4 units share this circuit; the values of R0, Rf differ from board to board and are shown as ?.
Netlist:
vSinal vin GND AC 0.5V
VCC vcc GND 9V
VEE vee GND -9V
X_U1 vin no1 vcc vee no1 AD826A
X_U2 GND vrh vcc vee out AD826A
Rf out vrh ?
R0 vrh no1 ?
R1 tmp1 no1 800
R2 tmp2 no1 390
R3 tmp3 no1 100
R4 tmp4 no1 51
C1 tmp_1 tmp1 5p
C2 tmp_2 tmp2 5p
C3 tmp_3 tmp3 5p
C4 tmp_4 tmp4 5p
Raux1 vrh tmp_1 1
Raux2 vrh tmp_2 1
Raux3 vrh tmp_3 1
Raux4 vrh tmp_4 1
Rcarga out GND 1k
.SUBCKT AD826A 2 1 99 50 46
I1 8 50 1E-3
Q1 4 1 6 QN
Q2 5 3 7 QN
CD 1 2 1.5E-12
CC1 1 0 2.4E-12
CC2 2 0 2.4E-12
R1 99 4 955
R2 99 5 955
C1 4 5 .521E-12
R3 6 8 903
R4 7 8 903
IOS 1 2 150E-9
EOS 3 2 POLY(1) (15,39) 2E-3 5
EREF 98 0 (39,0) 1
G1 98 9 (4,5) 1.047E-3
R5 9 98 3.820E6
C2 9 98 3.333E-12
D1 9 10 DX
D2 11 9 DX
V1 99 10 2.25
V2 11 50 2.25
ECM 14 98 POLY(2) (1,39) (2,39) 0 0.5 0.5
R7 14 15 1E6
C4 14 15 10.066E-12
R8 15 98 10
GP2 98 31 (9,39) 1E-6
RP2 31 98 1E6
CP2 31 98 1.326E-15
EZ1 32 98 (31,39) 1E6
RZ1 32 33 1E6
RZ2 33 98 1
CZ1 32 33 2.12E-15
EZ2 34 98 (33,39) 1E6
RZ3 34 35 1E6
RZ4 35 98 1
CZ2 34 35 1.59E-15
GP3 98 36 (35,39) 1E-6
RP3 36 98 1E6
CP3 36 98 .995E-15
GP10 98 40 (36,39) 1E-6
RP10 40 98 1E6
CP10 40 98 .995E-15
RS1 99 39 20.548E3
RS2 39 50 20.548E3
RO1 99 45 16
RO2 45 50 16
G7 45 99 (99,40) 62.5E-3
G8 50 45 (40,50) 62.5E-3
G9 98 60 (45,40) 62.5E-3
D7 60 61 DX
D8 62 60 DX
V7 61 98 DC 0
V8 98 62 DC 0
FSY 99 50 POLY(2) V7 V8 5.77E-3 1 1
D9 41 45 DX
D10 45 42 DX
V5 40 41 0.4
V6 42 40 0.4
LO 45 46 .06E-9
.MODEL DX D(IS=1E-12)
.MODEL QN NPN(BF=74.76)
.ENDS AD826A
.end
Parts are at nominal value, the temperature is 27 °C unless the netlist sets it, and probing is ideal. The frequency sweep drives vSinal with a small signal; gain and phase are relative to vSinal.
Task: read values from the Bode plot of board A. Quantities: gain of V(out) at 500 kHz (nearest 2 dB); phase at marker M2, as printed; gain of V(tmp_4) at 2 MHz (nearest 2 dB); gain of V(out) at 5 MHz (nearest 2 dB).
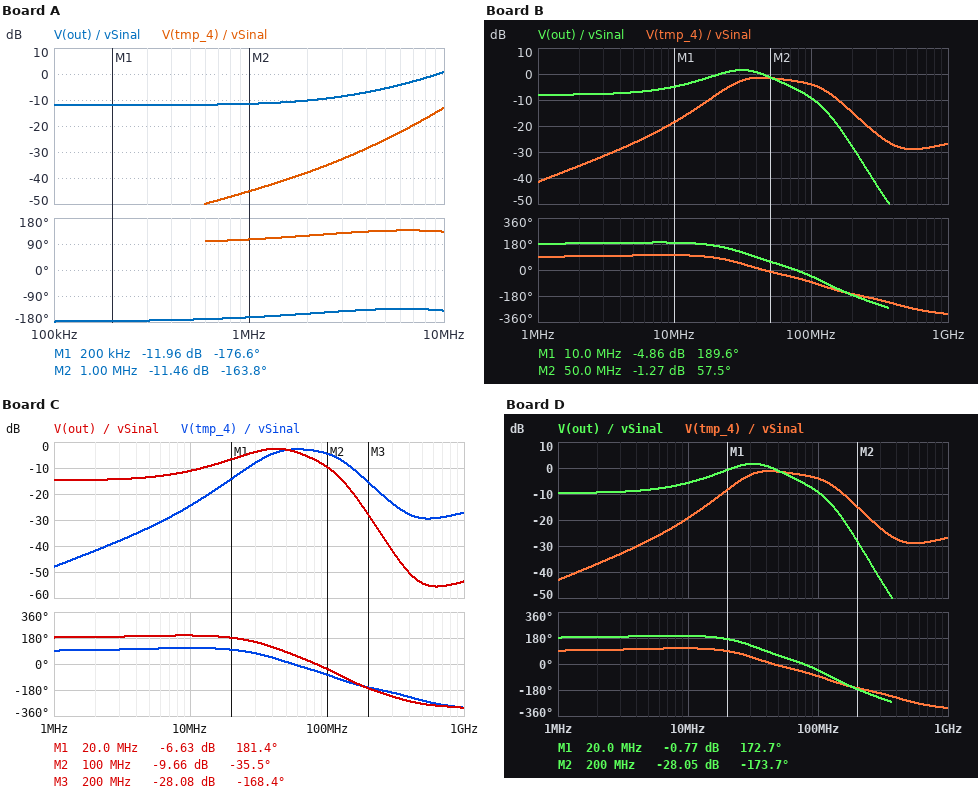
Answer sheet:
-12 dB
-163.8 deg
-38 dB
-6 dB
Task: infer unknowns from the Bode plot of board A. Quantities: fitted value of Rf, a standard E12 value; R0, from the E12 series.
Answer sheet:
680 Ω
2.7 kΩ
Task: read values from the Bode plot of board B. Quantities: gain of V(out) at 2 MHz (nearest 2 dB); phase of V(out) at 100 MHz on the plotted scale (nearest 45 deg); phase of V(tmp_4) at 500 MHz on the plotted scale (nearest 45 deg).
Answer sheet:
-8 dB
-45 deg
-270 deg
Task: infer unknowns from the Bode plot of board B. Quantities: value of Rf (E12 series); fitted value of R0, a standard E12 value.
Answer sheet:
270 Ω
680 Ω
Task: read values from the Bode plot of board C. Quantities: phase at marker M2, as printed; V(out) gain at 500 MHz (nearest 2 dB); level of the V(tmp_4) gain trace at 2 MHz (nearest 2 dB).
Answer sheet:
-35.5 deg
-54 dB
-42 dB
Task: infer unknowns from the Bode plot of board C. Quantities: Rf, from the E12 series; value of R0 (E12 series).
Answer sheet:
150 Ω
820 Ω
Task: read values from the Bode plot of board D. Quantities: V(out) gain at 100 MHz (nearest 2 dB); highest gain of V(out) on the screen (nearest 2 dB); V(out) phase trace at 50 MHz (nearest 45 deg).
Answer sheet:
-10 dB
2 dB
45 deg
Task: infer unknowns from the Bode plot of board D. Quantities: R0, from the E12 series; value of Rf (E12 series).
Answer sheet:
820 Ω
270 Ω
